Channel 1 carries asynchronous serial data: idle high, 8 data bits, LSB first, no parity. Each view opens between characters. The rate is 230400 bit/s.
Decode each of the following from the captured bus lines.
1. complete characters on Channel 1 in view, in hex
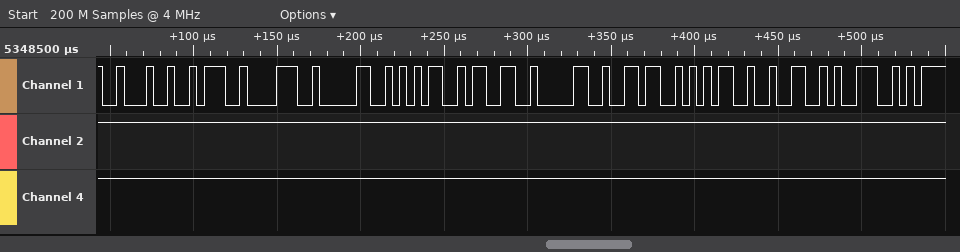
22, 3A, 38, 30, 35, 33, 30, 36, 35, 32, 39
